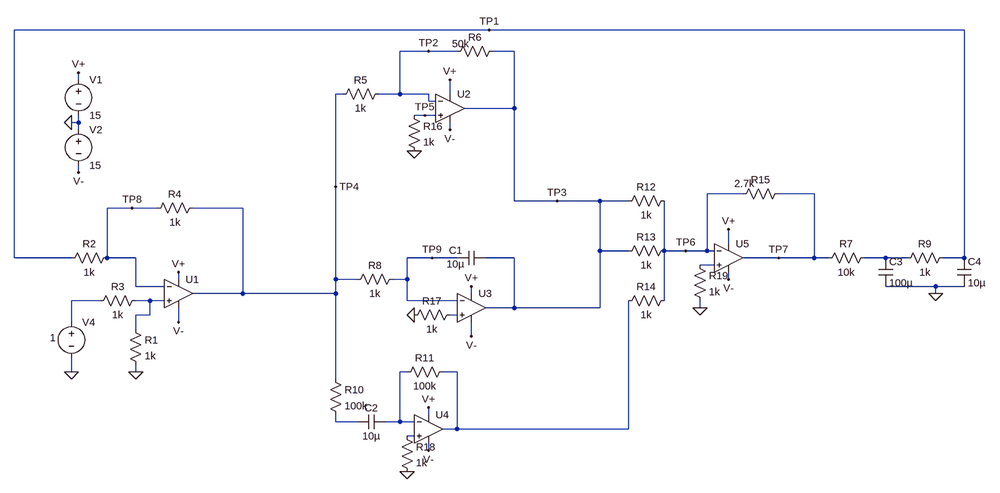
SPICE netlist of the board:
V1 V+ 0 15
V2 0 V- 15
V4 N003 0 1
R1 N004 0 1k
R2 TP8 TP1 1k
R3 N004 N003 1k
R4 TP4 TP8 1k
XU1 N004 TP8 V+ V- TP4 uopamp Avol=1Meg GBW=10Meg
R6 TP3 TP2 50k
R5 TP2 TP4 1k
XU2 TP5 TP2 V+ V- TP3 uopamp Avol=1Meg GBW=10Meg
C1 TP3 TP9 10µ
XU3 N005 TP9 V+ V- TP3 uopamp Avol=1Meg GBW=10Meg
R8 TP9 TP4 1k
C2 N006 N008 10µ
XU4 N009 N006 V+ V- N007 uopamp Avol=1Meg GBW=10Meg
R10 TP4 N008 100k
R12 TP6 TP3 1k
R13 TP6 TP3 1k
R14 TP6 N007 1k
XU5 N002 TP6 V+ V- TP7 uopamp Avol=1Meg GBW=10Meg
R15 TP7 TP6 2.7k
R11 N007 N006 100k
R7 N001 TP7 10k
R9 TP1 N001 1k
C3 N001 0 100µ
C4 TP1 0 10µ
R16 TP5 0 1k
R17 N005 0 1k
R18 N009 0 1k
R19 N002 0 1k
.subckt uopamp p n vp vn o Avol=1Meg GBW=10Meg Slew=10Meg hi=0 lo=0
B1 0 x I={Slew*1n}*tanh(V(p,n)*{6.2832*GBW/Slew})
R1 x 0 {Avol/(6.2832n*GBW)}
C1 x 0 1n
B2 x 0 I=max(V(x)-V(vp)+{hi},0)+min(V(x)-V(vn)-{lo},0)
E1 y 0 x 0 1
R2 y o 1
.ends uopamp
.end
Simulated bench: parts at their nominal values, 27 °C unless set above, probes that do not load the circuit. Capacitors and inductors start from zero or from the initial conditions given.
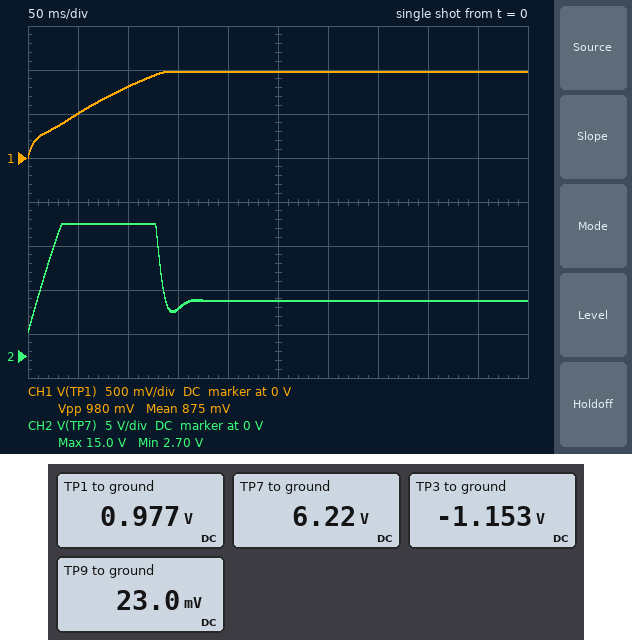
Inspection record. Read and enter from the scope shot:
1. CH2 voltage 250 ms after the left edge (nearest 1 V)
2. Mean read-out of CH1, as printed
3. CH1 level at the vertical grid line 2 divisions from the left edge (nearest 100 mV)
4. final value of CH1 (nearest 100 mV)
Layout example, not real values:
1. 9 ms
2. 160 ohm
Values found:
1. 6 V
2. 875 mV
3. 800 mV
4. 1.0 V
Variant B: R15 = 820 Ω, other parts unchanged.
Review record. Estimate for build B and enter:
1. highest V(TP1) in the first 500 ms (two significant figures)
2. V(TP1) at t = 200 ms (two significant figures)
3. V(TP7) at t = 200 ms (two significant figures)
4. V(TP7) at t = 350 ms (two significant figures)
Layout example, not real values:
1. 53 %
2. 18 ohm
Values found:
1. 930 mV
2. 920 mV
3. 6.4 V
4. 5.7 V
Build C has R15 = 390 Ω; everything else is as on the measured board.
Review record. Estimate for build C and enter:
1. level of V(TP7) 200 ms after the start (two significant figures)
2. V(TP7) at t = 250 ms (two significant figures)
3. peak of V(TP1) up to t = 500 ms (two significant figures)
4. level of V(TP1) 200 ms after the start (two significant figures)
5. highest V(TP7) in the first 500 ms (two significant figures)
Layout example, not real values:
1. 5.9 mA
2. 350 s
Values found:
1. 8.6 V
2. 6.7 V
3. 870 mV
4. 720 mV
5. 9.0 V
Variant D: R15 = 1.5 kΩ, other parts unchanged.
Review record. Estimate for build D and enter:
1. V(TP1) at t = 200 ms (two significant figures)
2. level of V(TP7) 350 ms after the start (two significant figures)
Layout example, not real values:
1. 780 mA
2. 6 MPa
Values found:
1. 960 mV
2. 6.0 V
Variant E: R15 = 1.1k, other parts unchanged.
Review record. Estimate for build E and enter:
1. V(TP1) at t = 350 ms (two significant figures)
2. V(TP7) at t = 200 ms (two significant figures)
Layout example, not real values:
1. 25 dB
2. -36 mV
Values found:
1. 950 mV
2. 5.9 V
